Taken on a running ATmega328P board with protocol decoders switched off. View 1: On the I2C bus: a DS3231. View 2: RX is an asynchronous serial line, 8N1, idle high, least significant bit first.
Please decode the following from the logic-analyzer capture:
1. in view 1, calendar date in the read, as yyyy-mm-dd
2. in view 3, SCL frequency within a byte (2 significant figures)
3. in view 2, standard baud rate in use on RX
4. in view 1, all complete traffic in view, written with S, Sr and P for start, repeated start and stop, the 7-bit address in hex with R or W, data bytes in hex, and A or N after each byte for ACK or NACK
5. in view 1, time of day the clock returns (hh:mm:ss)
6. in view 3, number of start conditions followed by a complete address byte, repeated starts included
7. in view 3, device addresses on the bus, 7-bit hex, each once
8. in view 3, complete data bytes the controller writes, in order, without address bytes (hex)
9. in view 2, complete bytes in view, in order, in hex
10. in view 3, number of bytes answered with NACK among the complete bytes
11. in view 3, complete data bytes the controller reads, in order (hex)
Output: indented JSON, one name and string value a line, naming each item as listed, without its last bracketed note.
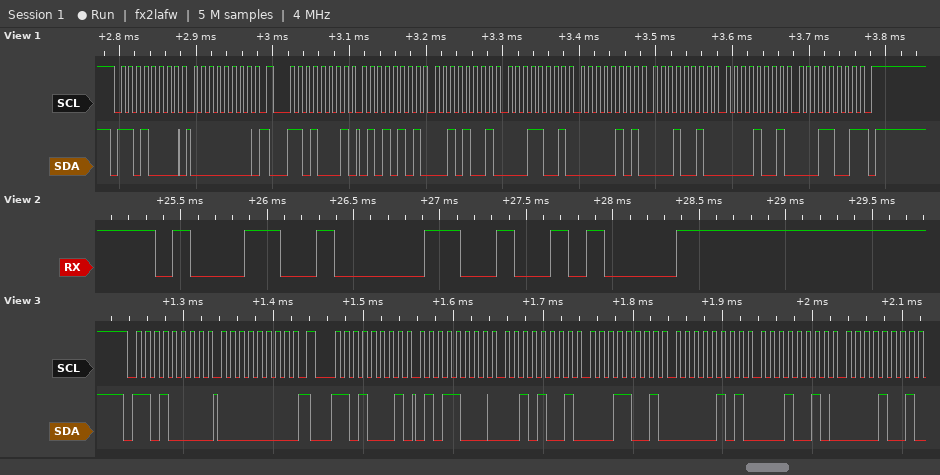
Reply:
{
  "in view 1, calendar date in the read, as yyyy-mm-dd": "2019-09-12",
  "in view 3, SCL frequency within a byte": "100 kHz",
  "in view 2, standard baud rate in use on RX": "9600 baud",
  "in view 1, all complete traffic in view, written with S, Sr and P for start, repeated start and stop, the 7-bit address in hex with R or W, data bytes in hex, and A or N after each byte for ACK or NACK": "S 68W A 00 A Sr 68R A 55 A 29 A 19 A 05 A 12 A 09 A 19 N P",
  "in view 1, time of day the clock returns": "19:29:55",
  "in view 3, number of start conditions followed by a complete address byte, repeated starts included": "2",
  "in view 3, device addresses on the bus, 7-bit hex, each once": "0x68",
  "in view 3, complete data bytes the controller writes, in order, without address bytes": "00",
  "in view 2, complete bytes in view, in order, in hex": "0x31 0x30 0x0A",
  "in view 3, number of bytes answered with NACK among the complete bytes": "0",
  "in view 3, complete data bytes the controller reads, in order": "58 29 19 05 12 09"
}
